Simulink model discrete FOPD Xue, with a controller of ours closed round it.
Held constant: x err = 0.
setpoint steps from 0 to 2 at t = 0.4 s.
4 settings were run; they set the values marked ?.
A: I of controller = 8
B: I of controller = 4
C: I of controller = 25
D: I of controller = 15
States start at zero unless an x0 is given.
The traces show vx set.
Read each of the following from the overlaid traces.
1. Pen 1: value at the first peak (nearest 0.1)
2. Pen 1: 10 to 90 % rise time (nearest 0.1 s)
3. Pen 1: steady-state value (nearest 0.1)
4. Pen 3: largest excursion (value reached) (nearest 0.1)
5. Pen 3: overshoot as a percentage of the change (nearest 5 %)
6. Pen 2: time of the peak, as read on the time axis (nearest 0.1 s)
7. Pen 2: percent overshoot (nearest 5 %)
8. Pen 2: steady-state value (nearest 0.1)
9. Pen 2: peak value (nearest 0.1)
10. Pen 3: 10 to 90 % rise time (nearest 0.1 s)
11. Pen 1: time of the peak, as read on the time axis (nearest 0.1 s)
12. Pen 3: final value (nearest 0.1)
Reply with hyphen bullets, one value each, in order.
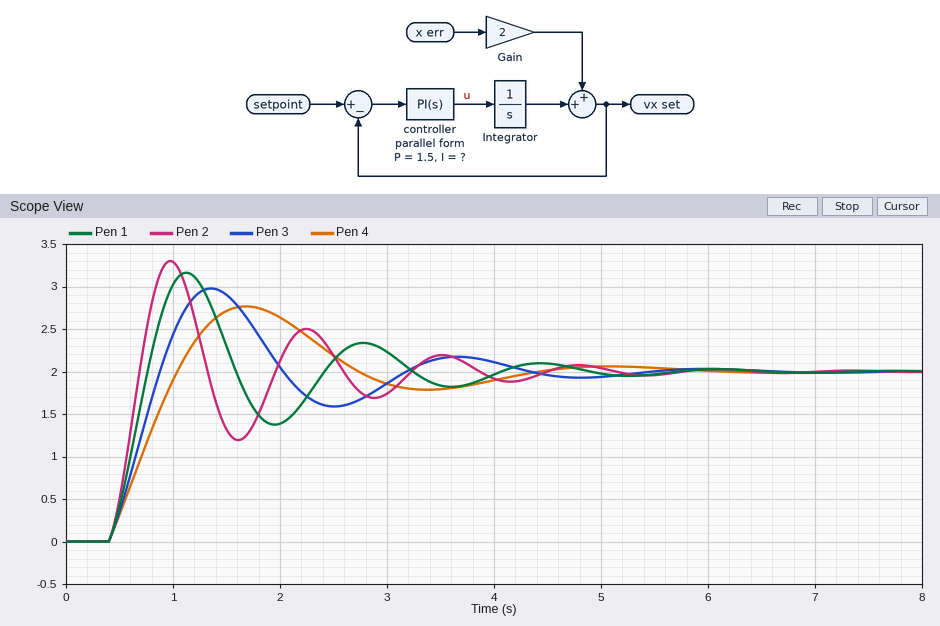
- 3.2
- 0.3 s
- 2.0
- 3.0
- 50 %
- 1.0 s
- 65 %
- 2.0
- 3.3
- 0.4 s
- 1.1 s
- 2.0
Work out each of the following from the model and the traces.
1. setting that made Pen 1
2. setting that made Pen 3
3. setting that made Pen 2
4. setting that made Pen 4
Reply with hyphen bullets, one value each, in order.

- D
- A
- C
- B
